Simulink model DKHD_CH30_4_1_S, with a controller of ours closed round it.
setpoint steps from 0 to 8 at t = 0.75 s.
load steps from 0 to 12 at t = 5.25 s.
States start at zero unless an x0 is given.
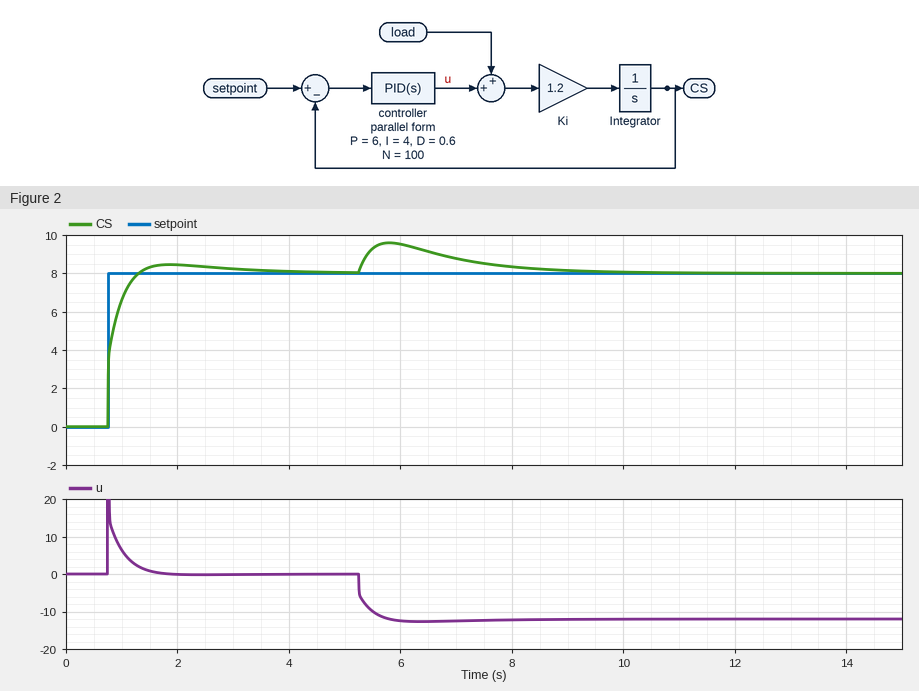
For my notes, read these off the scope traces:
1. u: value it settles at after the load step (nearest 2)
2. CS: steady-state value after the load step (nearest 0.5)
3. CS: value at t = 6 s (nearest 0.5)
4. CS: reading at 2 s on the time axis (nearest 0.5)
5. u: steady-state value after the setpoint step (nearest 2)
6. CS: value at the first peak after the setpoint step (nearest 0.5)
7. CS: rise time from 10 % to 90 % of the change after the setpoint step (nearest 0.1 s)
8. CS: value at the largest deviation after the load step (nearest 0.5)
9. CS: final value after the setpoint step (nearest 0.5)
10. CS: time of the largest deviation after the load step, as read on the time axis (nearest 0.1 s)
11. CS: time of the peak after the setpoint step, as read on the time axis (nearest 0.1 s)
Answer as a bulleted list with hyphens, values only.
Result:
- -12
- 8.0
- 9.5
- 8.5
- 0
- 8.5
- 0.3 s
- 9.5
- 8.0
- 5.8 s
- 1.9 s
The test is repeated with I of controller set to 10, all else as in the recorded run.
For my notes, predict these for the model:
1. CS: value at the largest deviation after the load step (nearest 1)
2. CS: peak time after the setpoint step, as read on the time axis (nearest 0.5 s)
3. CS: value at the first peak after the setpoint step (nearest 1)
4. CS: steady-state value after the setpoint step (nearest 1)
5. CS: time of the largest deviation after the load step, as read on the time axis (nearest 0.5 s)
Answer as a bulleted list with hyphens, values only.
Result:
- 9
- 1.5 s
- 9
- 8
- 5.5 s
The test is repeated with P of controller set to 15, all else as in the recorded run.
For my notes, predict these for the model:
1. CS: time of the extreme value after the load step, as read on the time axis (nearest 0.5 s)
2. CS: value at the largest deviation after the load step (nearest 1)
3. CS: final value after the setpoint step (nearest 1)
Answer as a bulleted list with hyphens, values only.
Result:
- 5.5 s
- 9
- 8
